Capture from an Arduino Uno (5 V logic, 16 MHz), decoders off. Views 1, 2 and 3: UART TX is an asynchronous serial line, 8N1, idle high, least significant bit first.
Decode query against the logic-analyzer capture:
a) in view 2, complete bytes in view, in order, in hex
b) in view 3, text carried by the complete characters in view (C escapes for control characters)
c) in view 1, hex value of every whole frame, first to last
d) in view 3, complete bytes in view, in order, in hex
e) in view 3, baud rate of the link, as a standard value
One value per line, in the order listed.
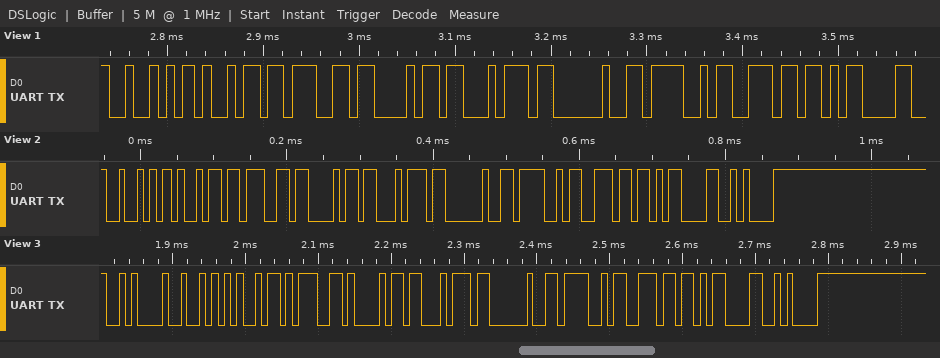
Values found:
0x52 0x69 0x67 0x68 0x74 0x20 0x4F 0x6E 0x0D 0x0A
"\nRight On\r\n"
52 69 67 68 74 20 4F 6E 0D
0A 52 69 67 68 74 20 4F 6E 0D 0A
115200 baud
